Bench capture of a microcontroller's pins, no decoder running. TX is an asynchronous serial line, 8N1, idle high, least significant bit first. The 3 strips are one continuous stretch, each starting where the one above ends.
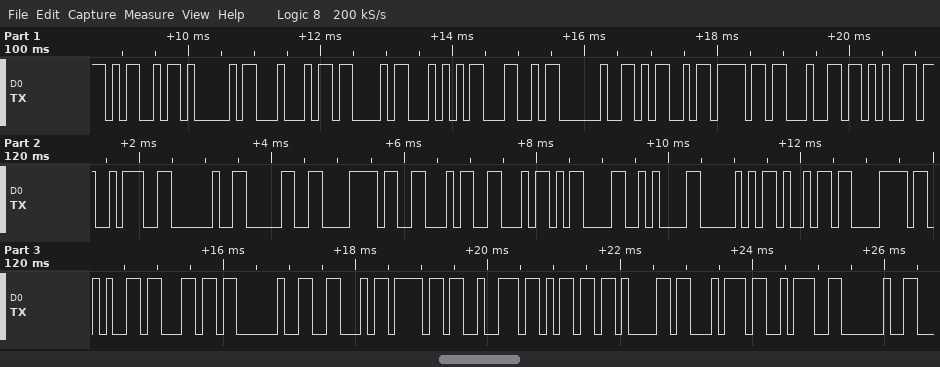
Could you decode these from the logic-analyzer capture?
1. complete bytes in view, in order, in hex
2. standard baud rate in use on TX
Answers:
4D 41 44 43 54 4C 20 4D 6F 64 65 3A 20 30 78 46 46 0D 0A 50 69 78 65 6C 20 46 6F 72 6D 61 74 3A 20
9600 baud
